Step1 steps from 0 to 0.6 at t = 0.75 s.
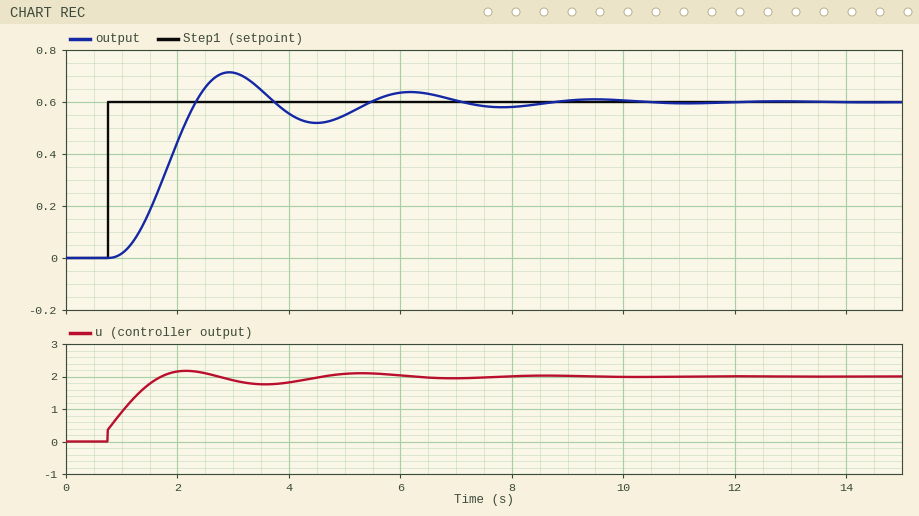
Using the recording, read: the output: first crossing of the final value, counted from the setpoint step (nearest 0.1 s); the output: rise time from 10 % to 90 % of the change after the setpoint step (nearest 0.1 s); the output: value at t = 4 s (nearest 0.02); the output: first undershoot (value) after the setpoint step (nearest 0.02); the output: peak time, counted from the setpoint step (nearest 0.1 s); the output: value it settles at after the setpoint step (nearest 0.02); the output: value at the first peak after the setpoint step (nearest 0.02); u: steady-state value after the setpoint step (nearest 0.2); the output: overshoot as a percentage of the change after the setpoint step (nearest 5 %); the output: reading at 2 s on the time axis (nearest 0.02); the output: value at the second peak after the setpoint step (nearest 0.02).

1.6 s
1.0 s
0.56
0.52
2.2 s
0.60
0.72
2.0
20 %
0.44
0.64
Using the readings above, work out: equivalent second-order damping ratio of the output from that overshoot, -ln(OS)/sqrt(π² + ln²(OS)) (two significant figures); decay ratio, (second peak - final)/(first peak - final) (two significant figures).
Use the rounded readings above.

0.46
0.33
